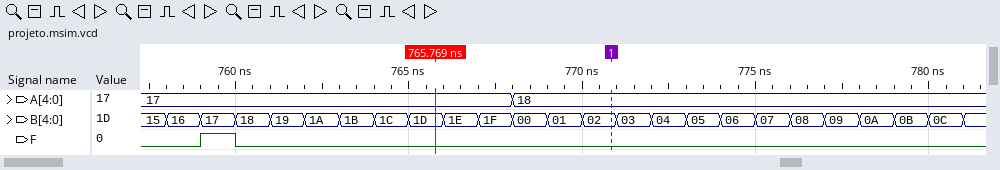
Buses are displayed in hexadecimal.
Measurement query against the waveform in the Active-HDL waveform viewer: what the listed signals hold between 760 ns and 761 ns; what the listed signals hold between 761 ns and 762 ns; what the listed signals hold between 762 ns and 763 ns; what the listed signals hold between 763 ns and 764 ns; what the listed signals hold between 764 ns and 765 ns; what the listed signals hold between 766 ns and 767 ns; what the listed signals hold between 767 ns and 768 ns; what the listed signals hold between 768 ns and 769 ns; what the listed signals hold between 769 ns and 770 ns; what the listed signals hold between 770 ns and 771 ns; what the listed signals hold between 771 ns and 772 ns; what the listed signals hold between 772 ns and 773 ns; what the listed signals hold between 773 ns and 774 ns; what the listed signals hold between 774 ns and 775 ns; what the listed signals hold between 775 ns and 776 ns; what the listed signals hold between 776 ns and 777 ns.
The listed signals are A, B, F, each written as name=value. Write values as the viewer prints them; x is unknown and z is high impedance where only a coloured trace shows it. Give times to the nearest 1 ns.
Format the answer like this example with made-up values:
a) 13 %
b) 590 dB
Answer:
a) A=17, B=18, F=0
b) A=17, B=19, F=0
c) A=17, B=1A, F=0
d) A=17, B=1B, F=0
e) A=17, B=1C, F=0
f) A=17, B=1E, F=0
g) A=17, B=1F, F=0
h) A=18, B=00, F=0
i) A=18, B=01, F=0
j) A=18, B=02, F=0
k) A=18, B=03, F=0
l) A=18, B=04, F=0
m) A=18, B=05, F=0
n) A=18, B=06, F=0
o) A=18, B=07, F=0
p) A=18, B=08, F=0
